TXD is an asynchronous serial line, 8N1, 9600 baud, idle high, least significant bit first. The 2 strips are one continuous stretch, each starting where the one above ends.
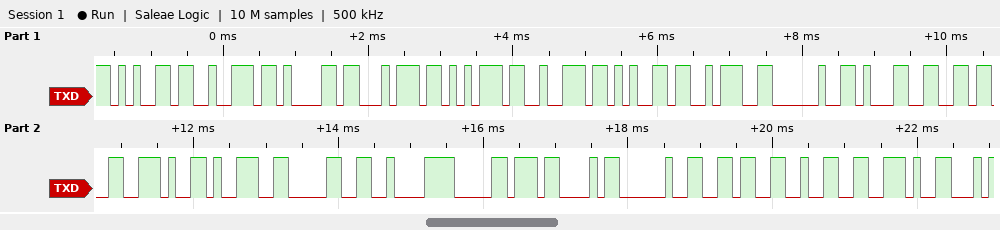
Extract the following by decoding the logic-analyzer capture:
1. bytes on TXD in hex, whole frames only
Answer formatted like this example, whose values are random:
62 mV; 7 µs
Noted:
65 72 61 74 75 72 65 3A 20 31 36 2E 39 30 C2 B0 43 20 36 32 2E
